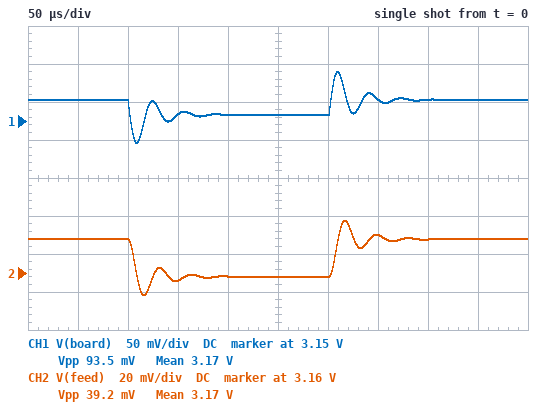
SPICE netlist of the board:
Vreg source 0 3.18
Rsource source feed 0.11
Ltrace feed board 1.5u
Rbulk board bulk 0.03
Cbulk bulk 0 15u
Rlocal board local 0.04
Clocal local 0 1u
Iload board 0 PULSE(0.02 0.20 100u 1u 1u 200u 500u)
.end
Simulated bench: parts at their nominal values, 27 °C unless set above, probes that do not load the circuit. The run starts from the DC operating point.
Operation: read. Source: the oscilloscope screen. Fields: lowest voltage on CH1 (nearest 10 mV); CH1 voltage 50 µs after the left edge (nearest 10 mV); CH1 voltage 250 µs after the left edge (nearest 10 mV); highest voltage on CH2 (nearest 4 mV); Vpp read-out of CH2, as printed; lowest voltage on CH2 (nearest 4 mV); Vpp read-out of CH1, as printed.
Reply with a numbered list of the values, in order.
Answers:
1. 3.12 V
2. 3.18 V
3. 3.16 V
4. 3.188 V
5. 39.2 mV
6. 3.148 V
7. 93.5 mV
